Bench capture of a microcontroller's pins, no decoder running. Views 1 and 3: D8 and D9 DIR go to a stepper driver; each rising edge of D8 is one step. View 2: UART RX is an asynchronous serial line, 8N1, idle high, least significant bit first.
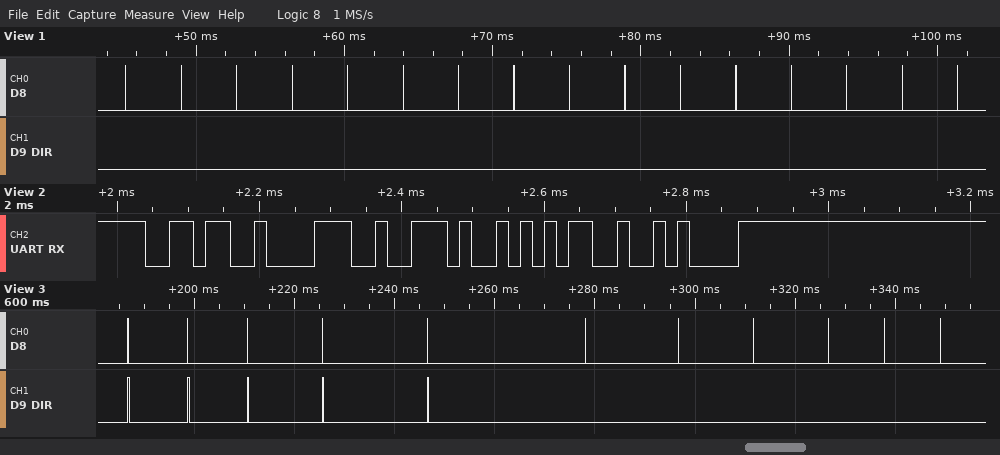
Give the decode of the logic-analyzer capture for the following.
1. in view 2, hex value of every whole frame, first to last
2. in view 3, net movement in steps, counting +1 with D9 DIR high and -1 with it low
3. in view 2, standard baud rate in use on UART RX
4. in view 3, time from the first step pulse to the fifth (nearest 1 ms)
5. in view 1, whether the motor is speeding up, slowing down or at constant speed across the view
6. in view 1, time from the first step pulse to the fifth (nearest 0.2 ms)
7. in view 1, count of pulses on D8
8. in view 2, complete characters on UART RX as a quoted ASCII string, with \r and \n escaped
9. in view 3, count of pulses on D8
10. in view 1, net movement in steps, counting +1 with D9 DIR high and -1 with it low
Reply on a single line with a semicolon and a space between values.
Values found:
0x36 0x38 0x2E 0x35 0x0A; -1; 57600 baud; 60 ms; constant speed; 15.0 ms; 16; "68.5\n"; 11; -16
